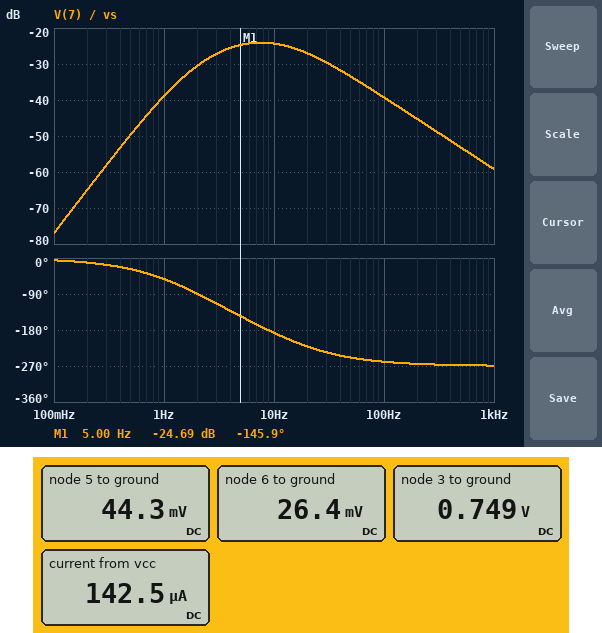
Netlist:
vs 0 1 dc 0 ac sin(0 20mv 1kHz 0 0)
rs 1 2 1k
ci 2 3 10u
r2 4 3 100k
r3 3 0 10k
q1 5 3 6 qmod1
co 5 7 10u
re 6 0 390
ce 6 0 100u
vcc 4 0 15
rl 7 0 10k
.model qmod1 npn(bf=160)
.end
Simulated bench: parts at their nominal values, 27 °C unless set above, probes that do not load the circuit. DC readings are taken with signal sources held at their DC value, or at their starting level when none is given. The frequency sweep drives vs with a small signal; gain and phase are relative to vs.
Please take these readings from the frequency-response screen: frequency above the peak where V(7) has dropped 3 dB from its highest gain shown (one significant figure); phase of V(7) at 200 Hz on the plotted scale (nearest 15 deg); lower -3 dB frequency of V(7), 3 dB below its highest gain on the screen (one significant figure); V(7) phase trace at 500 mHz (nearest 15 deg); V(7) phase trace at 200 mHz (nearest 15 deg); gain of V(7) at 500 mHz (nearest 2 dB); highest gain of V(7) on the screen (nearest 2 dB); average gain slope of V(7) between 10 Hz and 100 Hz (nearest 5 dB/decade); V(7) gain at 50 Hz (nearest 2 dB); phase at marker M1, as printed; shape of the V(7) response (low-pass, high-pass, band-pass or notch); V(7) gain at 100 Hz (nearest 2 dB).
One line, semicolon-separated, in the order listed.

20 Hz; -270 deg; 3 Hz; -30 deg; -15 deg; -50 dB; -24 dB; -15 dB/decade; -34 dB; -145.9 deg; band-pass; -40 dB
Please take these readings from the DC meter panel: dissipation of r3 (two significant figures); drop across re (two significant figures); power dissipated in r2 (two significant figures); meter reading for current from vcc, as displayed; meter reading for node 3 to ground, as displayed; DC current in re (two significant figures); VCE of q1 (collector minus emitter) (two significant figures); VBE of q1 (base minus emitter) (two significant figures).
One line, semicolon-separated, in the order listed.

56 µW; 26 mV; 2.0 mW; 142.5 µA; 0.749 V; 68 µA; 18 mV; 720 mV
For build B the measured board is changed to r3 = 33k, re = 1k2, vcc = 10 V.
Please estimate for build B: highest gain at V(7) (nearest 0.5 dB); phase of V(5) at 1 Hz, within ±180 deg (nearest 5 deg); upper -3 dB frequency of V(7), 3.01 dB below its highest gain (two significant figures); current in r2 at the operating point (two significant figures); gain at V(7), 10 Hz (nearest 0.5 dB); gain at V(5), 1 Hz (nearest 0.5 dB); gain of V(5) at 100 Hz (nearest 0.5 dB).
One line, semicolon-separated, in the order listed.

-22.5 dB; -135 deg; 17 Hz; 92 µA; -23.5 dB; -25.5 dB; -39.0 dB
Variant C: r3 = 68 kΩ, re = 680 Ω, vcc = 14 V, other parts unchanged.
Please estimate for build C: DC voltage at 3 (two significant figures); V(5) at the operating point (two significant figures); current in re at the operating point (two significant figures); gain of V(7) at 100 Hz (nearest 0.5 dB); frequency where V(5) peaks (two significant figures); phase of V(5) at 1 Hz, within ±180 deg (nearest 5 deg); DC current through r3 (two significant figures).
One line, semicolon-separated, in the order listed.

820 mV; 99 mV; 120 µA; -38.0 dB; 5.8 Hz; -120 deg; 12 µA
